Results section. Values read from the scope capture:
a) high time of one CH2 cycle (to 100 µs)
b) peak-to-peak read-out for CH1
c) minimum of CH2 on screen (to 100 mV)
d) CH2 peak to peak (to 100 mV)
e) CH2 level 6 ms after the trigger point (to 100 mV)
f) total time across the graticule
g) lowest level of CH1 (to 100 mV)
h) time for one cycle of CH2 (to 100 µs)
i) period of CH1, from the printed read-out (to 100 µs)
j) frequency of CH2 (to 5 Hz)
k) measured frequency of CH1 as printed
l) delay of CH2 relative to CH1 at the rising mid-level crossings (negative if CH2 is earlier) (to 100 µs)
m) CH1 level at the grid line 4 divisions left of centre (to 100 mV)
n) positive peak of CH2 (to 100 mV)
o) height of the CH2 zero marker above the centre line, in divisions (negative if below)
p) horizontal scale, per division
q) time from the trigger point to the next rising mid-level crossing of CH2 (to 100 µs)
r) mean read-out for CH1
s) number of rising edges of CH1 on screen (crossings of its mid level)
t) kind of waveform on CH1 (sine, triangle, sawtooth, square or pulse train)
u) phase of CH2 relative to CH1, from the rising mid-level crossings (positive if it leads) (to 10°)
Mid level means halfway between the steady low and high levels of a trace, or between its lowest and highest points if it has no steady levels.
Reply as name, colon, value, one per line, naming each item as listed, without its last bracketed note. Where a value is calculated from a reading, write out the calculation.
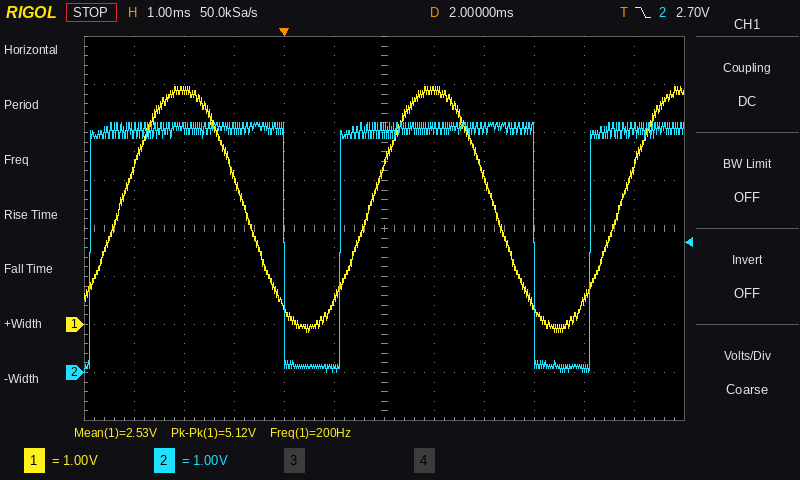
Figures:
high time of one CH2 cycle: 3.9 ms
peak-to-peak read-out for CH1: 5.12 V
minimum of CH2 on screen: 0.0 V
CH2 peak to peak: 5.2 V − (0.0 V) = 5.2 V
CH2 level 6 ms after the trigger point: 100 mV
total time across the graticule: 12 ms
lowest level of CH1: -200 mV
time for one cycle of CH2: 5.0 ms
period of CH1, from the printed read-out: 1 / 200 Hz ≈ 5.0 ms
frequency of CH2: 1 / 5.0 ms ≈ 200 Hz
measured frequency of CH1 as printed: 200 Hz
delay of CH2 relative to CH1 at the rising mid-level crossings (negative if CH2 is earlier): -600 µs
CH1 level at the grid line 4 divisions left of centre: 4.9 V
positive peak of CH2: 5.2 V
height of the CH2 zero marker above the centre line, in divisions: -3.0 div
horizontal scale, per division: 1 ms
time from the trigger point to the next rising mid-level crossing of CH2: 1.1 ms
mean read-out for CH1: 2.53 V
number of rising edges of CH1 on screen: 3
kind of waveform on CH1: sine
phase of CH2 relative to CH1, from the rising mid-level crossings (positive if it leads): −360° × (-600 µs) / 5.0 ms ≈ +43.2°, so +40° to the nearest 10°
